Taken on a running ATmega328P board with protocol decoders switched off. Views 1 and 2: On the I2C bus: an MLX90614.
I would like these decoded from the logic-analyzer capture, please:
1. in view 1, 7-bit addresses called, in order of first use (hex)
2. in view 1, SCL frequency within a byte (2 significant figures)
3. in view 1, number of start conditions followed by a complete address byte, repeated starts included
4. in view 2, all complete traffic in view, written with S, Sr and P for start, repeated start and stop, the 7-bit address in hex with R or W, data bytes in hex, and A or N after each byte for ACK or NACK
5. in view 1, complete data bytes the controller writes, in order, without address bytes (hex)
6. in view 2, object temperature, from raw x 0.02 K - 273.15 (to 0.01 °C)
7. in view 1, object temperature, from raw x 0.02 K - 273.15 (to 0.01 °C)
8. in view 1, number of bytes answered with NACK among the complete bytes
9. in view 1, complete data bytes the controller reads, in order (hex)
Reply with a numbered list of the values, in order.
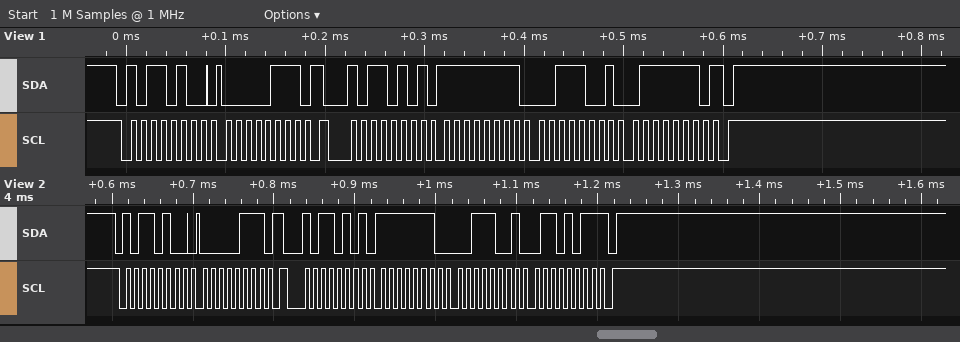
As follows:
1. 0x5A
2. 100 kHz
3. 2
4. S 5AW A 07 A Sr 5AR A FE A 39 A 6B N P
5. 07
6. 23.77 °C
7. 23.79 °C
8. 1
9. FF 39 7E
